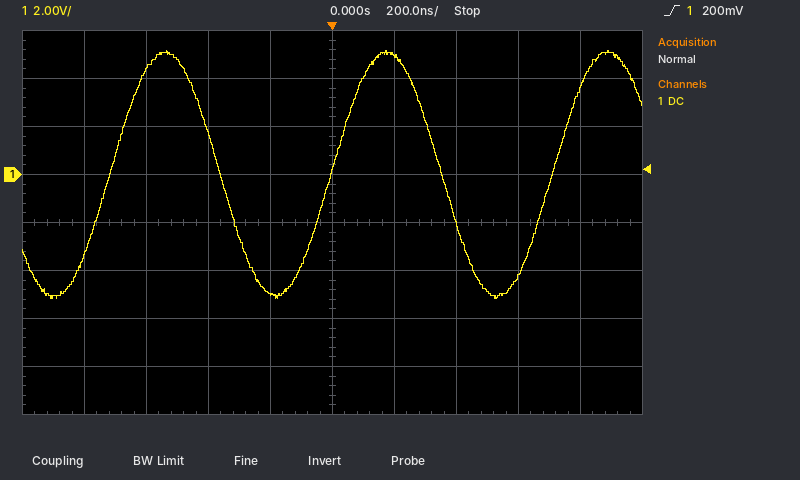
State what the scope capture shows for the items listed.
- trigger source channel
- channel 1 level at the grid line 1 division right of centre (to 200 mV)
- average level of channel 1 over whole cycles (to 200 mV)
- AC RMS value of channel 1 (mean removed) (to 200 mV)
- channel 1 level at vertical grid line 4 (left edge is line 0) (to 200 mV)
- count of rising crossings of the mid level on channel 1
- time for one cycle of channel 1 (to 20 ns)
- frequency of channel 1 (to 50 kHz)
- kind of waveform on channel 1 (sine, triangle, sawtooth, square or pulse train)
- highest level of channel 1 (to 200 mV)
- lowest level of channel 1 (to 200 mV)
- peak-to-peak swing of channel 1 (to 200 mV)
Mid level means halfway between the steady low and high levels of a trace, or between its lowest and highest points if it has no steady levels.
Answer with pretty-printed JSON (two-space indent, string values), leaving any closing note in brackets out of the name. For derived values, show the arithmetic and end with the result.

{
  "trigger source channel": "channel 1",
  "channel 1 level at the grid line 1 division right of centre": "5.0 V",
  "average level of channel 1 over whole cycles": "(5.2 V + (-5.2 V)) / 2 ≈ 0.0 V",
  "AC RMS value of channel 1 (mean removed)": "10.4 V / (2√2) ≈ 3.68 V, so 3.6 V to the nearest 200 mV",
  "channel 1 level at vertical grid line 4 (left edge is line 0)": "-5.0 V",
  "count of rising crossings of the mid level on channel 1": "3",
  "time for one cycle of channel 1": "720 ns",
  "frequency of channel 1": "1 / 720 ns ≈ 1.39 MHz, so 1.40 MHz to the nearest 50 kHz",
  "kind of waveform on channel 1": "sine",
  "highest level of channel 1": "5.2 V",
  "lowest level of channel 1": "-5.2 V",
  "peak-to-peak swing of channel 1": "5.2 V − (-5.2 V) = 10.4 V"
}
